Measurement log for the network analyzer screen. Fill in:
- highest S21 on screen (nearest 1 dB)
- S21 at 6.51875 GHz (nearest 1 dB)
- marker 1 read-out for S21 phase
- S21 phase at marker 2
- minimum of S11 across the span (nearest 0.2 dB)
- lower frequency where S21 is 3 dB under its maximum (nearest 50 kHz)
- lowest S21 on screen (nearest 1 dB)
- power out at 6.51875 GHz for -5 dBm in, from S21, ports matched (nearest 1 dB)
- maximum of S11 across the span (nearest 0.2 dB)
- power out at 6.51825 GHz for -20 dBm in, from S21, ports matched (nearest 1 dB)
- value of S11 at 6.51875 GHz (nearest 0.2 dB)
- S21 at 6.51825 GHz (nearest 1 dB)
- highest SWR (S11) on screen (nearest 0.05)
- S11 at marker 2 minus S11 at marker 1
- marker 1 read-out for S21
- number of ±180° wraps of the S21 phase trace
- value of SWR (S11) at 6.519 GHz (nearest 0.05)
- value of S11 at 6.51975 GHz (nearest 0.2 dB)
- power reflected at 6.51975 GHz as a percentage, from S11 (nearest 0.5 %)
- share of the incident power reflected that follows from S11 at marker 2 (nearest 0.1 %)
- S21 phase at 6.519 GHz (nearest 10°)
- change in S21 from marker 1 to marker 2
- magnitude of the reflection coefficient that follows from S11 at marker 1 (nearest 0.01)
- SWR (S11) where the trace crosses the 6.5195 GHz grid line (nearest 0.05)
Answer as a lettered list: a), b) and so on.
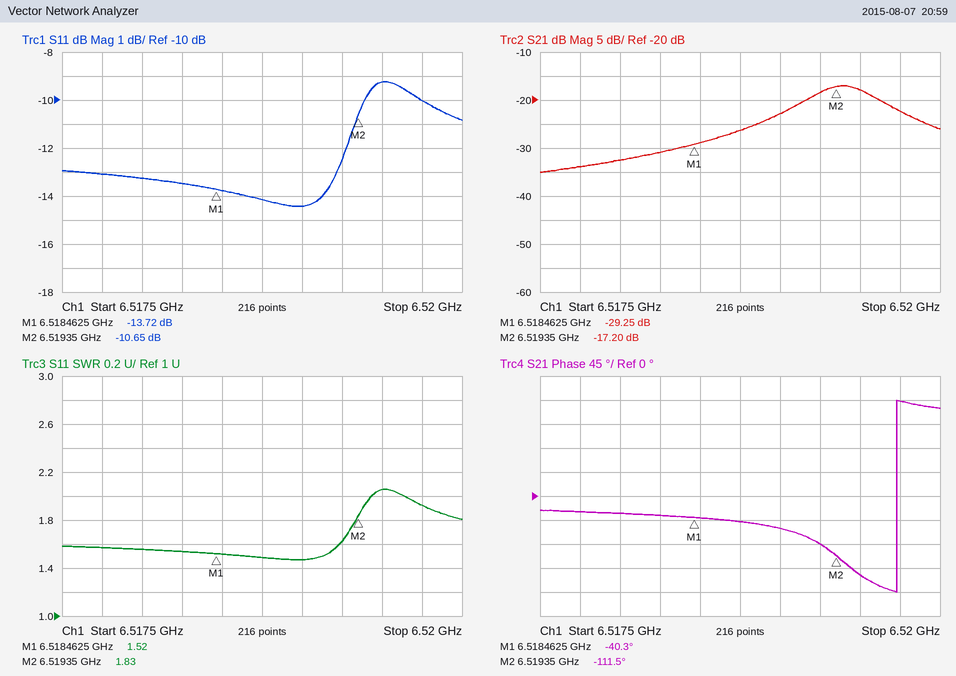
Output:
a) -17 dB
b) -26 dB
c) -40.3°
d) -111.5°
e) -14.4 dB
f) 6.51915 GHz
g) -35 dB
h) -31 dBm
i) -9.2 dB
j) -51 dBm
k) -14.2 dB
l) -31 dB
m) 2.05
n) 3.07 dB
o) -29.25 dB
p) 1
q) 1.45
r) -10.0 dB
s) 10.0 %
t) 8.6 %
u) -60°
v) 12.05 dB
w) 0.21
x) 2.05
